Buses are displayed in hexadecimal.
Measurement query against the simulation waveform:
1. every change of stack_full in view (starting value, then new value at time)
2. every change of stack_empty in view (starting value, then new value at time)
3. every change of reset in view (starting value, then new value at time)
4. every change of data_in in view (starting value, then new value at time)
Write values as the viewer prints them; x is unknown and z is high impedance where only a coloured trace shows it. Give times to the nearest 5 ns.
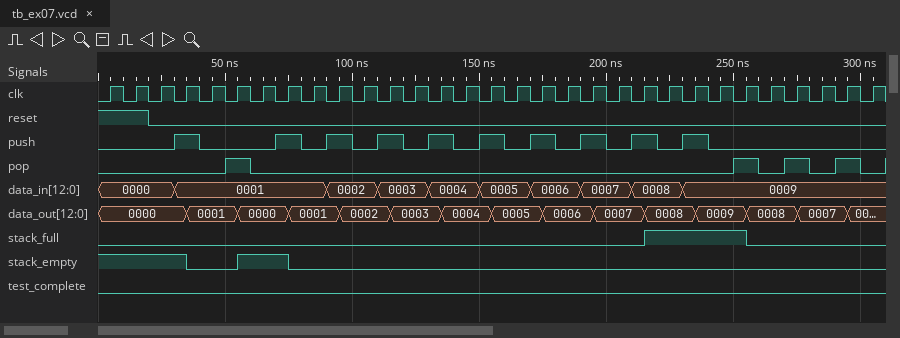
0, 1 at 215 ns, 0 at 255 ns
1, 0 at 35 ns, 1 at 55 ns, 0 at 75 ns
1, 0 at 20 ns
0000, 0001 at 30 ns, 0002 at 90 ns, 0003 at 110 ns, 0004 at 130 ns, 0005 at 150 ns, 0006 at 170 ns, 0007 at 190 ns, 0008 at 210 ns, 0009 at 230 ns
